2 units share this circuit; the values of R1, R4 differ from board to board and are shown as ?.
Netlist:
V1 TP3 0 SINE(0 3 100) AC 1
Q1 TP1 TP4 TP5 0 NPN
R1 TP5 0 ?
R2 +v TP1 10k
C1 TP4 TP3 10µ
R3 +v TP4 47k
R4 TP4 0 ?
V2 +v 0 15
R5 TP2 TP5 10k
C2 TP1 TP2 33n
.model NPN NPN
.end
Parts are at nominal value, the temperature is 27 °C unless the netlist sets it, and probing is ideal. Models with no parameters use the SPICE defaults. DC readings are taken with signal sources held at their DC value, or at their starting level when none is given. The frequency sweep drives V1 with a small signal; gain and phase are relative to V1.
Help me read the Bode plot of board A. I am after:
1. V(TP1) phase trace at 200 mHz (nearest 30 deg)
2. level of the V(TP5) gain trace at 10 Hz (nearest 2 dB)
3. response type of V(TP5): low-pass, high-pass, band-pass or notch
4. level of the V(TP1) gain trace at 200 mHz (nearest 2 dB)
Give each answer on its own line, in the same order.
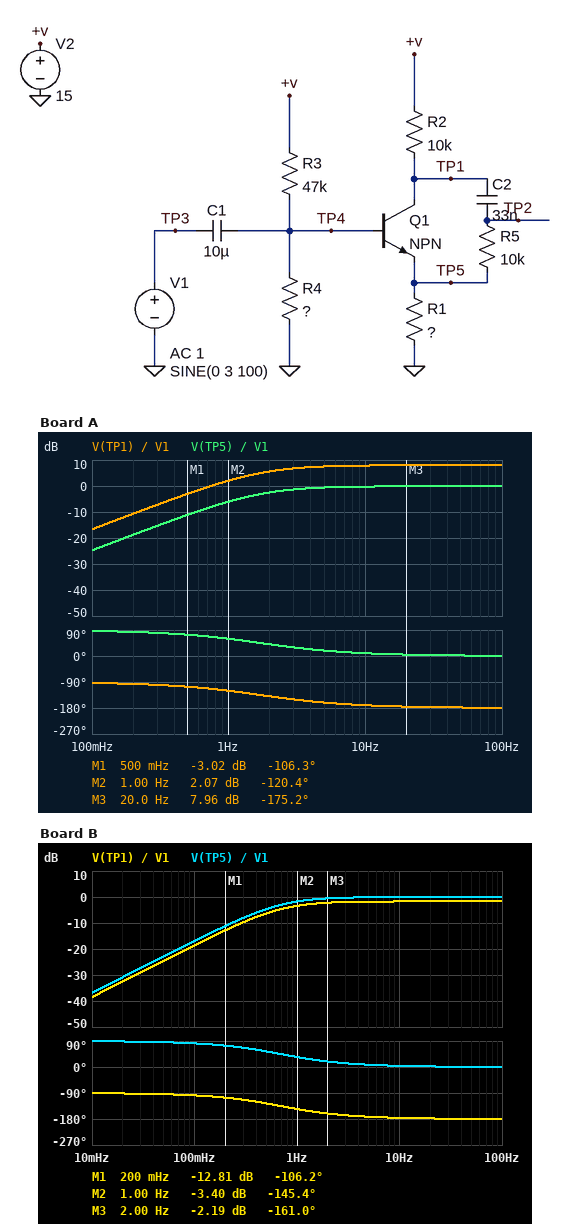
-90 deg
0 dB
high-pass
-10 dB
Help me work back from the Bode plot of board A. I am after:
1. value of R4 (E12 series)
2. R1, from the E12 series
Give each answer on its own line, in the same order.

12 kΩ
3.9 kΩ
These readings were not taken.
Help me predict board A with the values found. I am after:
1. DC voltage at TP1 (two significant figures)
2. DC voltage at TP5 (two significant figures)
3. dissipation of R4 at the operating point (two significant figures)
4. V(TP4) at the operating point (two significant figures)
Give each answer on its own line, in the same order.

9.3 V
2.2 V
750 µW
3.0 V
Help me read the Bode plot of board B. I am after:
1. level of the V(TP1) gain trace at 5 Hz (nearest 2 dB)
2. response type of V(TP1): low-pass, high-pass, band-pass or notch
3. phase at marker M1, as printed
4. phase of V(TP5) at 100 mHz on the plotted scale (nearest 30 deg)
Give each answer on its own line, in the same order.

-2 dB
high-pass
-106.2 deg
90 deg
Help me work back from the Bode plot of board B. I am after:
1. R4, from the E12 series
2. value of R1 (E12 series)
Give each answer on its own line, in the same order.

47 kΩ
12 kΩ
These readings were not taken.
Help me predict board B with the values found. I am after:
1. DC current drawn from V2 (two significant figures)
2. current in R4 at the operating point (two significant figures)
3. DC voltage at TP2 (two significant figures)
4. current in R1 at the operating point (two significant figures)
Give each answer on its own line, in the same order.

710 µA
160 µA
6.6 V
550 µA
